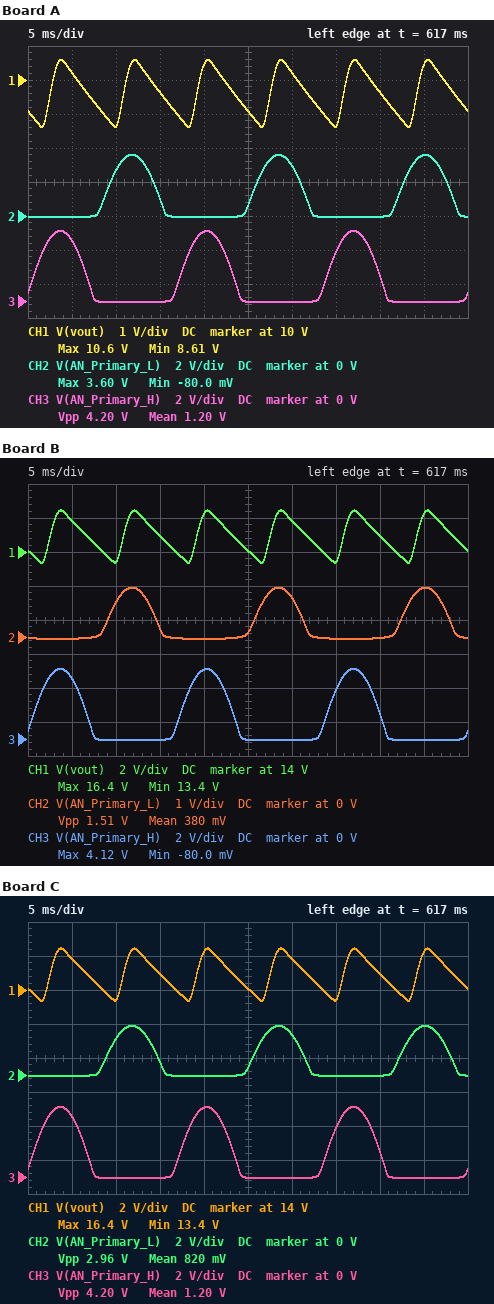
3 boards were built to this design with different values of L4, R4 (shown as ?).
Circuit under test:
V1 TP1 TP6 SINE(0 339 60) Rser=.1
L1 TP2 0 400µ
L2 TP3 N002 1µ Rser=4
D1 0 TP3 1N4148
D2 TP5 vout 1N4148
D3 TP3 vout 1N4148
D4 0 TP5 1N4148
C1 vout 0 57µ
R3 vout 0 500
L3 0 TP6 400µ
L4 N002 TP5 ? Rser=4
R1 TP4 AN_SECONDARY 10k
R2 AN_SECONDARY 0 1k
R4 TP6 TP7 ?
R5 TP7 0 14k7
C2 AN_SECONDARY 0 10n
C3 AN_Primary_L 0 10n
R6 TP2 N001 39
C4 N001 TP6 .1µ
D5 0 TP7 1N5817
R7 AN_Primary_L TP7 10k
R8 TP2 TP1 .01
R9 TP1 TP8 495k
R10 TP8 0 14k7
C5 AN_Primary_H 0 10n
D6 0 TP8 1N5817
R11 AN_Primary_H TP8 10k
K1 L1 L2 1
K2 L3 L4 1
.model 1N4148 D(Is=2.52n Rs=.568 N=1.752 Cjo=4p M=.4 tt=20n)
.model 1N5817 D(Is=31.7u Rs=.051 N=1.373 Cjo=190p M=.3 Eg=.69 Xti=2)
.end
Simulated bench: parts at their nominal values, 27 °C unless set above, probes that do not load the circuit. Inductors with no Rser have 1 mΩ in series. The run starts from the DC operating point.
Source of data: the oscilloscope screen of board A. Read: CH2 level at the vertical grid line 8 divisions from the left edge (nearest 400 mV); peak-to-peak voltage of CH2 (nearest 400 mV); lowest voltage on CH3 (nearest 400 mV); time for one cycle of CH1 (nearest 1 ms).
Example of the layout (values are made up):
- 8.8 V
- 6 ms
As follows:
- 0 V
- 3.6 V
- 0 V
- 8 ms
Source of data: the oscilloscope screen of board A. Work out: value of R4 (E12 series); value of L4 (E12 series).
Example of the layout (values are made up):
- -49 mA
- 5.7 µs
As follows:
- 560 kΩ
- 330 nH
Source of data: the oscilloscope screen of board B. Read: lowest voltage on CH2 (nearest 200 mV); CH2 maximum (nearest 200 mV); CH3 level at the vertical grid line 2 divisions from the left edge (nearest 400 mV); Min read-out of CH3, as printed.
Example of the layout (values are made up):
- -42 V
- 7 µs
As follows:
- 0 V
- 1.4 V
- 0 V
- -80.0 mV
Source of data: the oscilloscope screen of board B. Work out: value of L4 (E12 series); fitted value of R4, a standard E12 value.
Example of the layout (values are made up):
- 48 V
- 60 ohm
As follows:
- 1.8 µH
- 1.2 MΩ
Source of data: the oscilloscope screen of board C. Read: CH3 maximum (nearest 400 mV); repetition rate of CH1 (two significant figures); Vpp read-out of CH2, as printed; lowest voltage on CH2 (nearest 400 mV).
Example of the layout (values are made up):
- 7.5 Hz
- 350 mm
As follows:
- 4.0 V
- 120 Hz
- 2.96 V
- 0 V
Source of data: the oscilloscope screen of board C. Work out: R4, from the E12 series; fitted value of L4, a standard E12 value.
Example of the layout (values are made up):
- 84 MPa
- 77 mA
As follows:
- 680 kΩ
- 1.8 µH
